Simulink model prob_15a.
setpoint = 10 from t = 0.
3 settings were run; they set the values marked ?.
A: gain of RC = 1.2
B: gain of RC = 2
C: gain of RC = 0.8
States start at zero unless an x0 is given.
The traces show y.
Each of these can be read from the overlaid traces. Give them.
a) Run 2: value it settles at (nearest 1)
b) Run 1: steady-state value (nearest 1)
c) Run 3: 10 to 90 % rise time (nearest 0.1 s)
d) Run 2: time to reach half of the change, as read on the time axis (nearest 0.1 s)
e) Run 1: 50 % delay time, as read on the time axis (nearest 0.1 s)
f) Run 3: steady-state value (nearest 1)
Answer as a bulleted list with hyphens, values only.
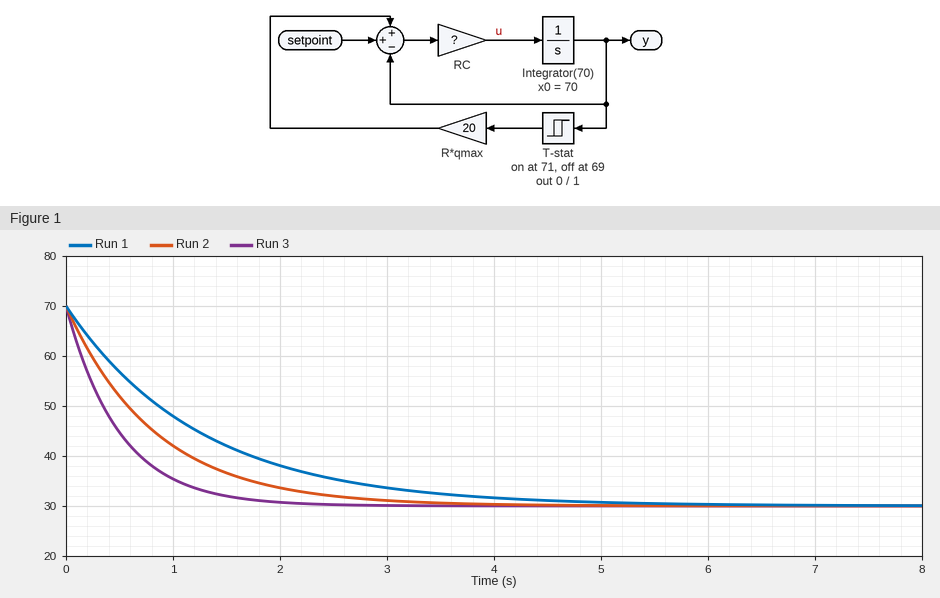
- 30
- 30
- 1.1 s
- 0.6 s
- 0.9 s
- 30
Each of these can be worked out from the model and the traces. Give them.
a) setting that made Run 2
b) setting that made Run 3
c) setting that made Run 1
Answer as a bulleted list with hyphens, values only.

- A
- B
- C
